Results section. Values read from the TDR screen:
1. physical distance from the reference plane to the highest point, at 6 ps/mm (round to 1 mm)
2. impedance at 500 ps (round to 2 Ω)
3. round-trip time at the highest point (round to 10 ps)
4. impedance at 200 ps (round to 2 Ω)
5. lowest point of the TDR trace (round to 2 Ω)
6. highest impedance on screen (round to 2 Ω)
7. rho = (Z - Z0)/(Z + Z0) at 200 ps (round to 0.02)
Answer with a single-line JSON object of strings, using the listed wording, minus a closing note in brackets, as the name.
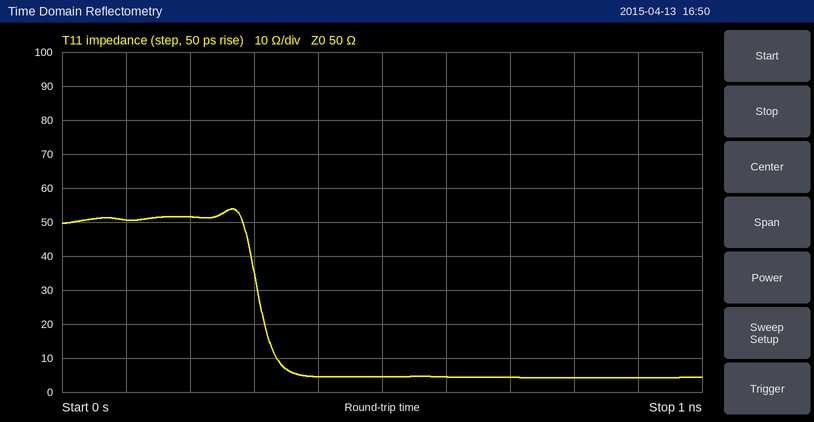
{"physical distance from the reference plane to the highest point, at 6 ps/mm": "22 mm", "impedance at 500 ps": "4 Ω", "round-trip time at the highest point": "270 ps", "impedance at 200 ps": "52 Ω", "lowest point of the TDR trace": "4 Ω", "highest impedance on screen": "54 Ω", "rho = (Z - Z0)/(Z + Z0) at 200 ps": "+0.02"}
